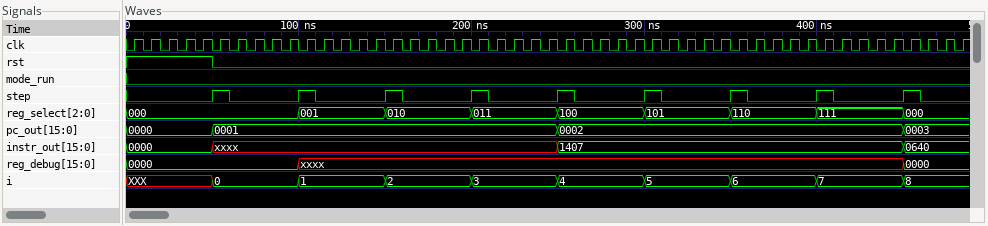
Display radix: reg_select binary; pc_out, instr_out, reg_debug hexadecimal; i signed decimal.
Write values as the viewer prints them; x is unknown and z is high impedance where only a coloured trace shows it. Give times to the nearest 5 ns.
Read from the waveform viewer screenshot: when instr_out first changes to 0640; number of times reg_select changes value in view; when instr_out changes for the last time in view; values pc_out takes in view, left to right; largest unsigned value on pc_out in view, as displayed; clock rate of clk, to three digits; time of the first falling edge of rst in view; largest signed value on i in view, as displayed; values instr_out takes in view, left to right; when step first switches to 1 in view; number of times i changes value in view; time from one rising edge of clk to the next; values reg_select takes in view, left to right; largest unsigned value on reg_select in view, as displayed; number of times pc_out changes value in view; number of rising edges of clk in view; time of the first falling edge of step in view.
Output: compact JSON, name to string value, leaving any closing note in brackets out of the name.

{"when instr_out first changes to 0640": "450 ns", "number of times reg_select changes value in view": "8", "when instr_out changes for the last time in view": "450 ns", "values pc_out takes in view, left to right": "0000, 0001, 0002, 0003", "largest unsigned value on pc_out in view, as displayed": "0003", "clock rate of clk, to three digits": "100 MHz", "time of the first falling edge of rst in view": "50 ns", "largest signed value on i in view, as displayed": "8", "values instr_out takes in view, left to right": "0000, xxxx, 1407, 0640", "when step first switches to 1 in view": "50 ns", "number of times i changes value in view": "9", "time from one rising edge of clk to the next": "10 ns", "values reg_select takes in view, left to right": "000, 001, 010, 011, 100, 101, 110, 111, 000", "largest unsigned value on reg_select in view, as displayed": "111", "number of times pc_out changes value in view": "3", "number of rising edges of clk in view": "49", "time of the first falling edge of step in view": "60 ns"}
